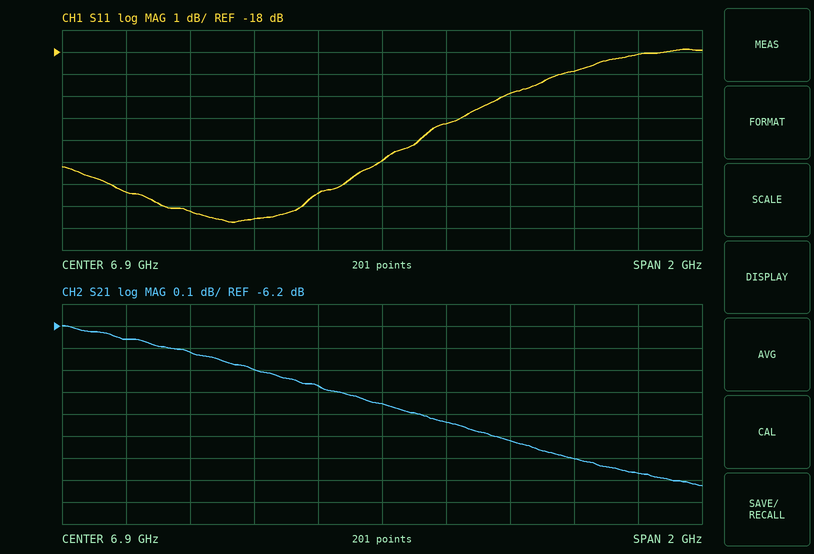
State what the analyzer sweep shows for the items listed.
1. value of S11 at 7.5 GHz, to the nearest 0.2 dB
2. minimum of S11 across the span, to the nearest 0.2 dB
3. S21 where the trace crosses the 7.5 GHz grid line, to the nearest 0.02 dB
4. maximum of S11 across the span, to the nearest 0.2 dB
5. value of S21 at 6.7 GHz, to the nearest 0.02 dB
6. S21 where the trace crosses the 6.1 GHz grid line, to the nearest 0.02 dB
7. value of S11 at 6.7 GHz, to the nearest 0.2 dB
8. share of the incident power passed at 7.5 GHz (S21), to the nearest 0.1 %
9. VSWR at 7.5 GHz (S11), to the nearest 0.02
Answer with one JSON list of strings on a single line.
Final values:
["-18.8 dB", "-25.8 dB", "-6.80 dB", "-17.8 dB", "-6.48 dB", "-6.26 dB", "-24.4 dB", "20.9 %", "1.26"]
